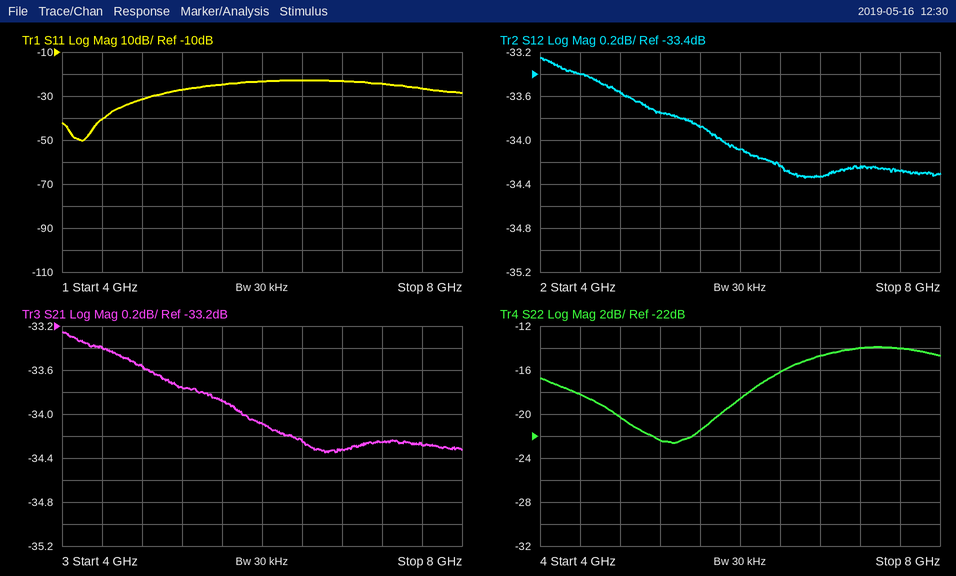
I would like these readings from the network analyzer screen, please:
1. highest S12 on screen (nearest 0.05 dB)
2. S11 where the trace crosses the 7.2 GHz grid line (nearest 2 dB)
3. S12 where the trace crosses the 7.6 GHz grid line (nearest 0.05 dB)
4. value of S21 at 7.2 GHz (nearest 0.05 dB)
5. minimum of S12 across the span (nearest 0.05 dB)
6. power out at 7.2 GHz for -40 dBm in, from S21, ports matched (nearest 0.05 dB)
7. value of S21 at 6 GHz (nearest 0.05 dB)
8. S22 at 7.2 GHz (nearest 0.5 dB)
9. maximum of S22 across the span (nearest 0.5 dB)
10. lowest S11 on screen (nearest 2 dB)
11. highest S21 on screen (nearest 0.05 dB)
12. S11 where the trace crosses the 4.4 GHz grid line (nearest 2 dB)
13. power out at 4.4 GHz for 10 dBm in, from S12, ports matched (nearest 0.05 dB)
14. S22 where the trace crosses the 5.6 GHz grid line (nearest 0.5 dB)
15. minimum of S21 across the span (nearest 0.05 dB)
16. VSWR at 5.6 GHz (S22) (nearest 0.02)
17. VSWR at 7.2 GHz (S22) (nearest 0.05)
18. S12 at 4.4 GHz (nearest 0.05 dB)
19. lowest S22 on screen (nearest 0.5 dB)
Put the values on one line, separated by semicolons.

-33.25 dB; -24 dB; -34.30 dB; -34.25 dB; -34.35 dB; -74.25 dBm; -34.10 dB; -14.0 dB; -14.0 dB; -50 dB; -33.25 dB; -40 dB; -23.40 dBm; -21.5 dB; -34.35 dB; 1.18; 1.50; -33.40 dB; -22.5 dB
